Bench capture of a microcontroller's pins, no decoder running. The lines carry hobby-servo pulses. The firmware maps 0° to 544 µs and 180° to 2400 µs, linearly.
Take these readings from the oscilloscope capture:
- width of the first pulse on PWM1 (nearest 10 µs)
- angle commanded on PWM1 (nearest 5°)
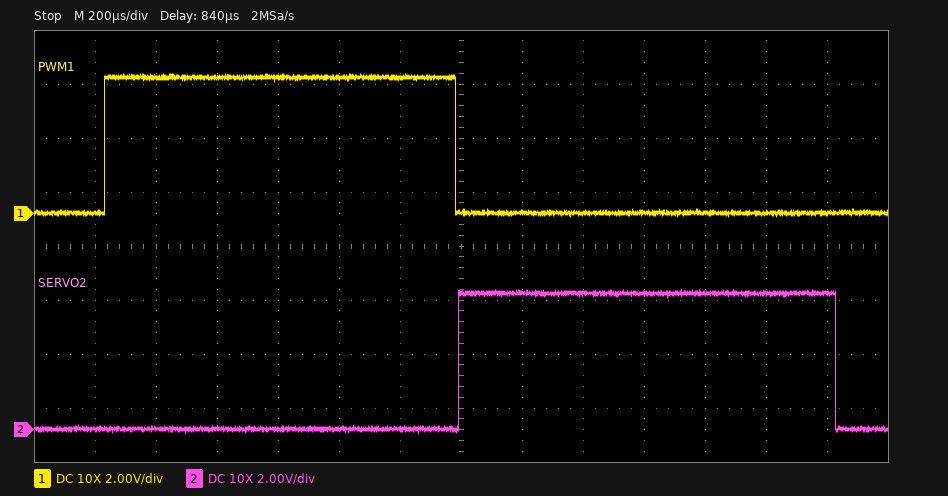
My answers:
1150 µs
60°
